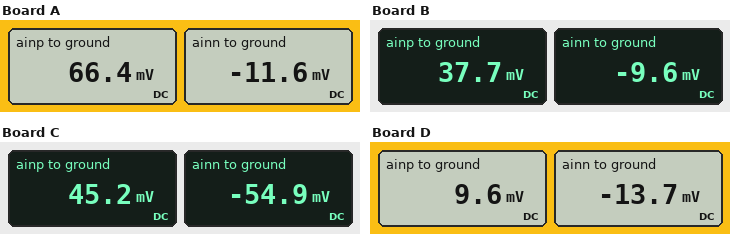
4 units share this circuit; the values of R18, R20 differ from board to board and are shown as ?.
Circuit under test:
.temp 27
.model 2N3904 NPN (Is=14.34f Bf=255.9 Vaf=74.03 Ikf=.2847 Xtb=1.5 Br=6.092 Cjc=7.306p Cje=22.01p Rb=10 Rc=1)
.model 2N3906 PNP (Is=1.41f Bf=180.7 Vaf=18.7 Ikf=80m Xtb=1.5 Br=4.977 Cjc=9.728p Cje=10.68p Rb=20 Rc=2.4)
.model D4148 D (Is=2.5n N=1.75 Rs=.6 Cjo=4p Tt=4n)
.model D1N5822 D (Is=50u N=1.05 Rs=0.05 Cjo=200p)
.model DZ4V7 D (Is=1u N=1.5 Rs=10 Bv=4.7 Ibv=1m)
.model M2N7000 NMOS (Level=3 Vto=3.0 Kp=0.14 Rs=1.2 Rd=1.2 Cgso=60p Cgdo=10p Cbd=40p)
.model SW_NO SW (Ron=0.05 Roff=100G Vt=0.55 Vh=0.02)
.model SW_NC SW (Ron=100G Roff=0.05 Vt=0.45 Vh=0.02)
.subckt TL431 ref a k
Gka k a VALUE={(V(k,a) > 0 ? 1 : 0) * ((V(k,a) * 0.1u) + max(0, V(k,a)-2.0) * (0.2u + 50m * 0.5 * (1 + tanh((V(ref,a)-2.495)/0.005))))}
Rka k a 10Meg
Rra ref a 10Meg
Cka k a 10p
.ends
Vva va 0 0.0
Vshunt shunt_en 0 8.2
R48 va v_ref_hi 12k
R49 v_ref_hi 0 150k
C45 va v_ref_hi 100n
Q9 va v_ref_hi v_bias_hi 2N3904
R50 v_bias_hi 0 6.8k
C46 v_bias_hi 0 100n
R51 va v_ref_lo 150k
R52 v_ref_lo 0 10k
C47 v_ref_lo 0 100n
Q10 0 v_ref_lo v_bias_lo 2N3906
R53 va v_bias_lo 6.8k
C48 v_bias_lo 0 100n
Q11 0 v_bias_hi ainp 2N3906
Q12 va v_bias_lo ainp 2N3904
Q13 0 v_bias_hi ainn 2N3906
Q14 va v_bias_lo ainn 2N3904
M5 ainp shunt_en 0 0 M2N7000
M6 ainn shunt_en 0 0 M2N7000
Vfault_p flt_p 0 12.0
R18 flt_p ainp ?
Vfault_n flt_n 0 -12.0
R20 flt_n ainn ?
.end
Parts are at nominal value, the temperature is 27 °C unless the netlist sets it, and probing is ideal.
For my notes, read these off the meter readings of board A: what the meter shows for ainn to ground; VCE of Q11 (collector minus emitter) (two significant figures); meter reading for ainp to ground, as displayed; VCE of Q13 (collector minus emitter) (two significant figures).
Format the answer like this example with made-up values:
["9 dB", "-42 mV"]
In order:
["-11.6 mV", "-66 mV", "66.4 mV", "12 mV"]
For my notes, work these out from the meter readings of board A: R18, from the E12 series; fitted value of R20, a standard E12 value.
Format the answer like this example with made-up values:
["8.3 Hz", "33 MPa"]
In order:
["680 Ω", "3.9 kΩ"]
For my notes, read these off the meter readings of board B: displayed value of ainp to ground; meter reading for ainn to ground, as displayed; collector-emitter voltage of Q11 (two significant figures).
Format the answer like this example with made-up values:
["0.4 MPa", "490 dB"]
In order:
["37.7 mV", "-9.6 mV", "-38 mV"]
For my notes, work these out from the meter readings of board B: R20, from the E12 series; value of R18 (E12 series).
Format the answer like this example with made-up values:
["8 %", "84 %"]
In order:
["4.7 kΩ", "1.2 kΩ"]
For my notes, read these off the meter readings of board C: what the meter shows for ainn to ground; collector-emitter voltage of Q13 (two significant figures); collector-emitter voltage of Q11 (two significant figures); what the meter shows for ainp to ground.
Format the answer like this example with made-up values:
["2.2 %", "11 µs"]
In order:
["-54.9 mV", "55 mV", "-45 mV", "45.2 mV"]
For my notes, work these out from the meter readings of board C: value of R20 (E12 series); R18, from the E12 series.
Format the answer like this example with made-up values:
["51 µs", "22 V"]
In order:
["820 Ω", "1 kΩ"]
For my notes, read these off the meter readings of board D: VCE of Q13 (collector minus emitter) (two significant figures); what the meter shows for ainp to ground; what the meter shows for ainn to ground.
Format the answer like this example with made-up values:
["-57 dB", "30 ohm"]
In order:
["14 mV", "9.6 mV", "-13.7 mV"]
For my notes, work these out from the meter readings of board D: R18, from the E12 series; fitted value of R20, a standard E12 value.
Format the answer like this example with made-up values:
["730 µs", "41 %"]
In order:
["4.7 kΩ", "3.3 kΩ"]
